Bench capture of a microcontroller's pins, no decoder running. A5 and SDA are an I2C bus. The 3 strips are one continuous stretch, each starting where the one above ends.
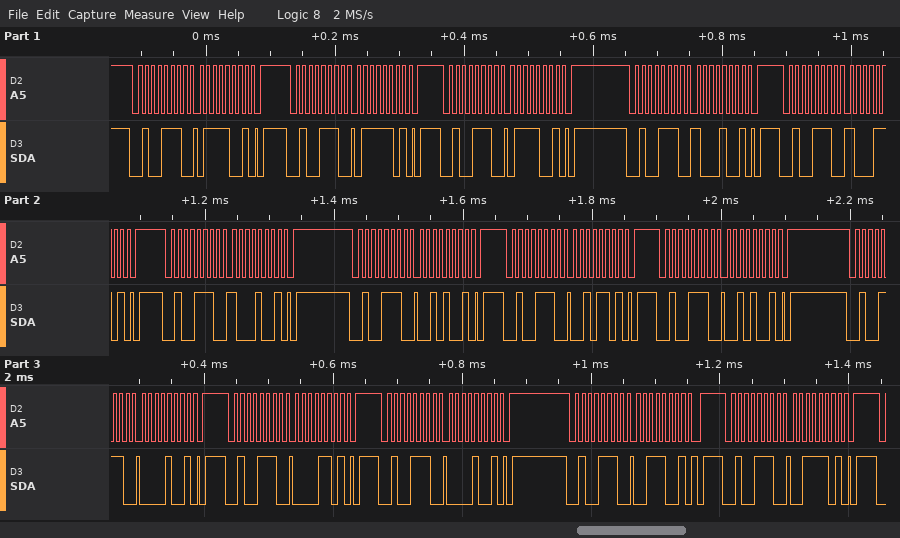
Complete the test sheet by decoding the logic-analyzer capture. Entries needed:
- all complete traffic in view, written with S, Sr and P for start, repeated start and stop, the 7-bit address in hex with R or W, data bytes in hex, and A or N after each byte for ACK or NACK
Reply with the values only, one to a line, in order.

S 27W A 79 A P S 27W A 7D A P S 27W A 79 A P S 27W A 89 A P S 27W A 8D A P S 27W A 89 A P S 27W A 29 A P S 27W A 2D A P S 27W A 29 A P S 27W A 09 A P S 27W A 0D A P S 27W A 09 A P S 27W A 39 A P S 27W A 3D A P
